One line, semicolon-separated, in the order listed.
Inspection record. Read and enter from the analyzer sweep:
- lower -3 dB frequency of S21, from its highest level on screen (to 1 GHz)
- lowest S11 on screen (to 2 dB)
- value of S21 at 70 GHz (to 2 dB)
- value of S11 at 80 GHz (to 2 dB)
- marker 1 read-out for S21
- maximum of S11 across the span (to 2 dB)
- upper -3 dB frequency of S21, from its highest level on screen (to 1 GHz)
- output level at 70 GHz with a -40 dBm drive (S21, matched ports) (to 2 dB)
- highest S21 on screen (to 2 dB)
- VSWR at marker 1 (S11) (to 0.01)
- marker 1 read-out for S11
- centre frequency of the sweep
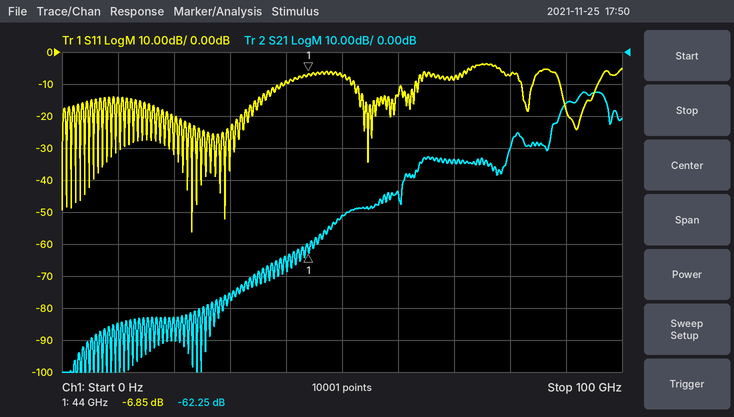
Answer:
92 GHz; -56 dB; -34 dB; -8 dB; -62.25 dB; -4 dB; 97 GHz; -74 dBm; -12 dB; 2.67; -6.85 dB; 50 GHz
